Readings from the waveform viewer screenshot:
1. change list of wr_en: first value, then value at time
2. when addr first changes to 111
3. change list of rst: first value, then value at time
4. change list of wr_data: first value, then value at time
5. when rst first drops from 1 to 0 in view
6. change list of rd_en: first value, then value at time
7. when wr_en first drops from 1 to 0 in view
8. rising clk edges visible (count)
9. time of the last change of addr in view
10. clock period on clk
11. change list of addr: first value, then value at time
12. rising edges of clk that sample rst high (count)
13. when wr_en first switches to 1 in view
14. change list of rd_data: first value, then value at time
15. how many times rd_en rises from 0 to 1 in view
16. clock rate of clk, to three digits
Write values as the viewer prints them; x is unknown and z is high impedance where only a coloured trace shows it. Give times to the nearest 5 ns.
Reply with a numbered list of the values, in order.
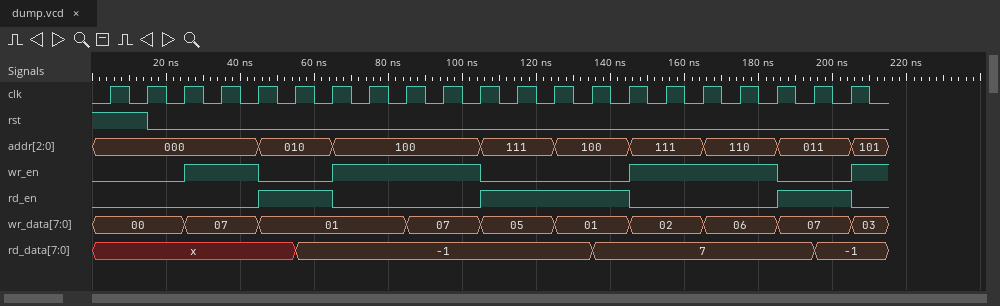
1. 0, 1 at 25 ns, 0 at 45 ns, 1 at 65 ns, 0 at 105 ns, 1 at 145 ns, 0 at 185 ns, 1 at 205 ns
2. 105 ns
3. 1, 0 at 15 ns
4. 00, 07 at 25 ns, 01 at 45 ns, 07 at 85 ns, 05 at 105 ns, 01 at 125 ns, 02 at 145 ns, 06 at 165 ns, 07 at 185 ns, 03 at 205 ns
5. 15 ns
6. 0, 1 at 45 ns, 0 at 65 ns, 1 at 105 ns, 0 at 145 ns, 1 at 185 ns, 0 at 205 ns
7. 45 ns
8. 21
9. 205 ns
10. 10 ns
11. 000, 010 at 45 ns, 100 at 65 ns, 111 at 105 ns, 100 at 125 ns, 111 at 145 ns, 110 at 165 ns, 011 at 185 ns, 101 at 205 ns
12. 2
13. 25 ns
14. x, -1 at 55 ns, 7 at 135 ns, -1 at 195 ns
15. 3
16. 100 MHz
